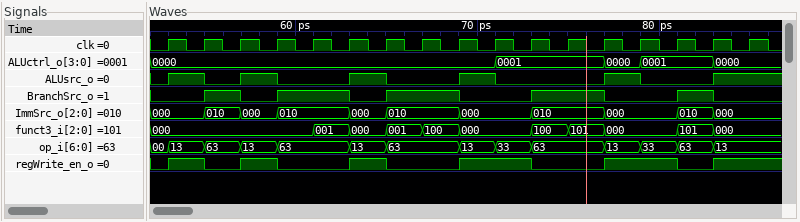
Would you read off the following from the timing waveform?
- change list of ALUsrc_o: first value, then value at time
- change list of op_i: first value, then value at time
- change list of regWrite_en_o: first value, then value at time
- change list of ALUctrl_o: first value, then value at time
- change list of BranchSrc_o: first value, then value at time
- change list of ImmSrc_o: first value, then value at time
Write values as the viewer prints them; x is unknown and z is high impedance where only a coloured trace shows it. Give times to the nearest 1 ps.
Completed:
0, 1 at 53 ps, 0 at 55 ps, 1 at 57 ps, 0 at 59 ps, 1 at 63 ps, 0 at 65 ps, 1 at 69 ps, 0 at 71 ps, 1 at 77 ps, 0 at 79 ps, 1 at 83 ps
00, 13 at 53 ps, 63 at 55 ps, 13 at 57 ps, 63 at 59 ps, 13 at 63 ps, 63 at 65 ps, 13 at 69 ps, 33 at 71 ps, 63 at 73 ps, 13 at 77 ps, 33 at 79 ps, 63 at 81 ps, 13 at 83 ps
0, 1 at 53 ps, 0 at 55 ps, 1 at 57 ps, 0 at 59 ps, 1 at 63 ps, 0 at 65 ps, 1 at 69 ps, 0 at 73 ps, 1 at 77 ps, 0 at 81 ps, 1 at 83 ps
0000, 0001 at 71 ps, 0000 at 77 ps, 0001 at 79 ps, 0000 at 83 ps
0, 1 at 55 ps, 0 at 57 ps, 1 at 59 ps, 0 at 63 ps, 1 at 65 ps, 0 at 69 ps, 1 at 73 ps, 0 at 77 ps, 1 at 81 ps, 0 at 83 ps
000, 010 at 55 ps, 000 at 57 ps, 010 at 59 ps, 000 at 63 ps, 010 at 65 ps, 000 at 69 ps, 010 at 73 ps, 000 at 77 ps, 010 at 81 ps, 000 at 83 ps
